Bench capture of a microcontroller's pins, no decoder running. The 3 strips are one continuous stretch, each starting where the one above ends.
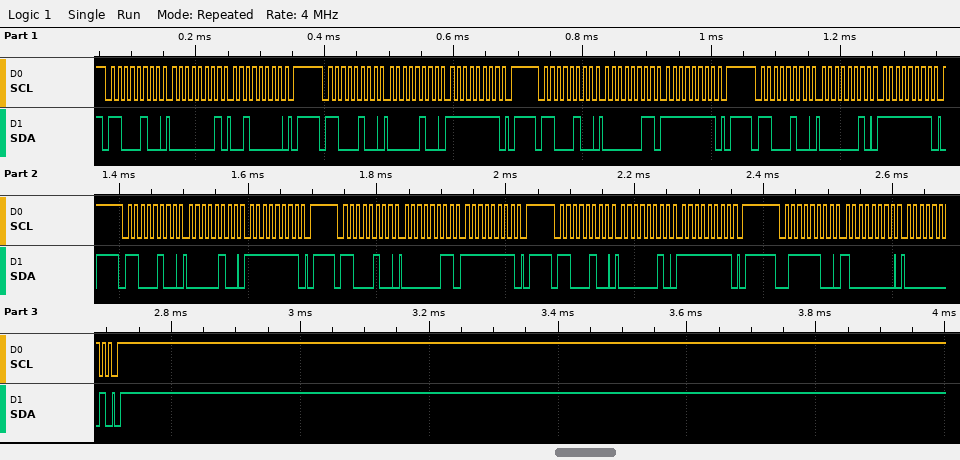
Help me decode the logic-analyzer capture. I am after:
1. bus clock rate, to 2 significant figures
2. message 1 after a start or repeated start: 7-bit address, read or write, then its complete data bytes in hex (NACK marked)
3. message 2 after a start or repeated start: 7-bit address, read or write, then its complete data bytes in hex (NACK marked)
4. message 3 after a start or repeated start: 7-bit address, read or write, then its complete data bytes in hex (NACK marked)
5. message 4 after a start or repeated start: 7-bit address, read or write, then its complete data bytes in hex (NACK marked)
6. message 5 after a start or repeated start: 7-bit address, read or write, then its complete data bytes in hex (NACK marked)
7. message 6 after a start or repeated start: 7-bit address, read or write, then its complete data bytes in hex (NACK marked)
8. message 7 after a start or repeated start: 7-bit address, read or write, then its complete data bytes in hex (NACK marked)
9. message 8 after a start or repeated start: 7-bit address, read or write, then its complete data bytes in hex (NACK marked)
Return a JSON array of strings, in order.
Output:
["100 kHz", "0x62 write: 01 20", "0x62 write: 04 FF", "0x62 write: 03 FF", "0x62 write: 02 FF", "0x62 write: 04 FF", "0x62 write: 03 FF", "0x62 write: 02 FF", "0x3E write: 80 01"]
